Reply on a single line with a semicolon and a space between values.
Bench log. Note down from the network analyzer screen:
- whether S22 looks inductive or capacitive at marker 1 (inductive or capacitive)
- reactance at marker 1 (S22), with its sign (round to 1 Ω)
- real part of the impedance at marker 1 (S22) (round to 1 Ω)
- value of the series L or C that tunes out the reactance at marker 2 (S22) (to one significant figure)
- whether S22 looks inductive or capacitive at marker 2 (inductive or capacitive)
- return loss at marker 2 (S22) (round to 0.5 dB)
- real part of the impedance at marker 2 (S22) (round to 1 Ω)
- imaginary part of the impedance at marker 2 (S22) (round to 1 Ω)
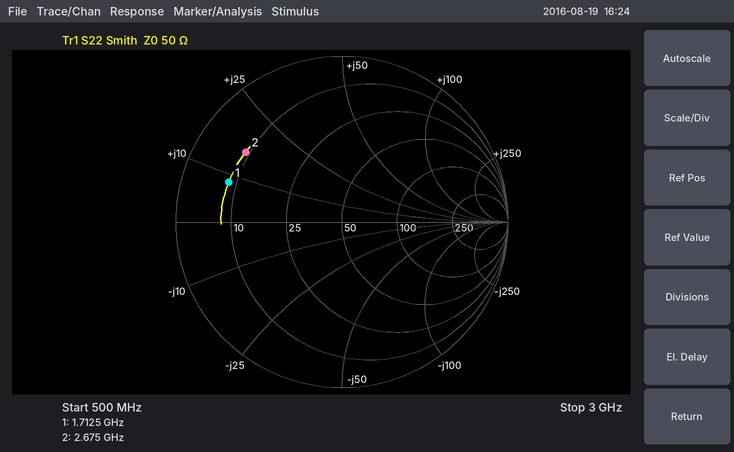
inductive; +8 Ω; 8 Ω; 4 pF; inductive; 3.0 dB; 9 Ω; +16 Ω
